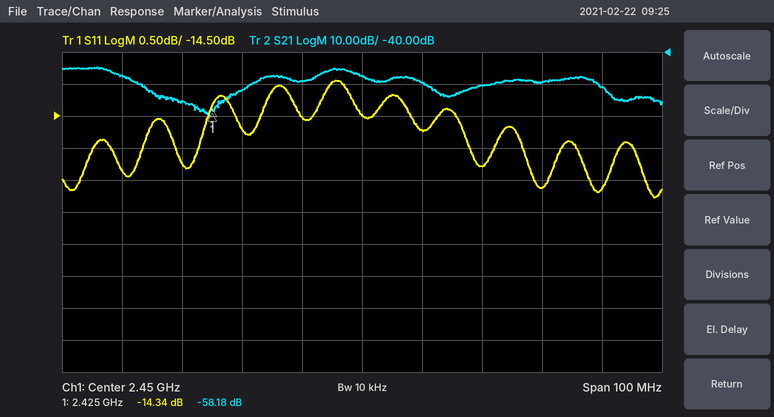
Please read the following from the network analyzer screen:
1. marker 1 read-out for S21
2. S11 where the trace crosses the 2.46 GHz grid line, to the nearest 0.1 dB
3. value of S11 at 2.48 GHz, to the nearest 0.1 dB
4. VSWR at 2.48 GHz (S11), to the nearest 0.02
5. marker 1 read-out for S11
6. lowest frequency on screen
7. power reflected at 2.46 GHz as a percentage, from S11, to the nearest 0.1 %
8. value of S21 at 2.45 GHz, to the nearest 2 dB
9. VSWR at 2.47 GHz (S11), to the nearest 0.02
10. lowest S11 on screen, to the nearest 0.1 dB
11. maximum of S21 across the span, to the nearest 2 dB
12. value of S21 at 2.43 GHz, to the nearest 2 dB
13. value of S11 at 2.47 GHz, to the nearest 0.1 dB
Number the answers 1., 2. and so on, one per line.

1. -58.18 dB
2. -14.7 dB
3. -15.6 dB
4. 1.40
5. -14.34 dB
6. 2.4 GHz
7. 3.4 %
8. -48 dB
9. 1.42
10. -15.8 dB
11. -44 dB
12. -52 dB
13. -15.3 dB
